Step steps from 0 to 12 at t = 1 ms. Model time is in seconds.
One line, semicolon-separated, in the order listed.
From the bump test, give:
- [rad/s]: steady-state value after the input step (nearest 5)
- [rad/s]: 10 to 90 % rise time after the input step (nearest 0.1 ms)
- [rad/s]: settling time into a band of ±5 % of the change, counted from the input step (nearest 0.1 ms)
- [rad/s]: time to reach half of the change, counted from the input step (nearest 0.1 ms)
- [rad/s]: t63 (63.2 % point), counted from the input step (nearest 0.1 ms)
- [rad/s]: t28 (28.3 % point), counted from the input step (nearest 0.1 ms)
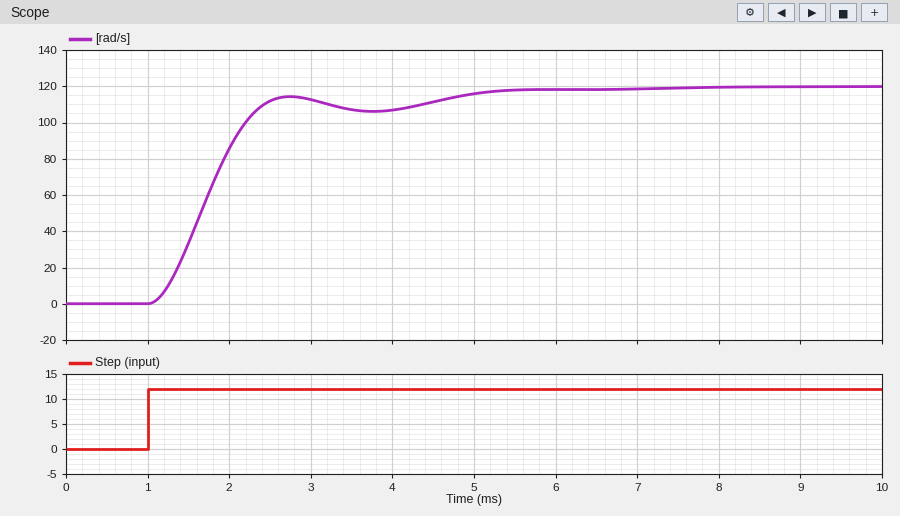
120; 1.1 ms; 3.8 ms; 0.7 ms; 0.9 ms; 0.5 ms
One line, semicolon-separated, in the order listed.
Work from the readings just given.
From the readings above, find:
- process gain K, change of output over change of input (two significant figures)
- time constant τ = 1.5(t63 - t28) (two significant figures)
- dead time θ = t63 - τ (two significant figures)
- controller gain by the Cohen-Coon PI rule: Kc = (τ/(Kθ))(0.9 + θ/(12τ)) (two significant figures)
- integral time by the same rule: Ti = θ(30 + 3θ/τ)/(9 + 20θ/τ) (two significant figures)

10; 0.60 ms; 0.30 ms; 0.19; 0.50 ms
